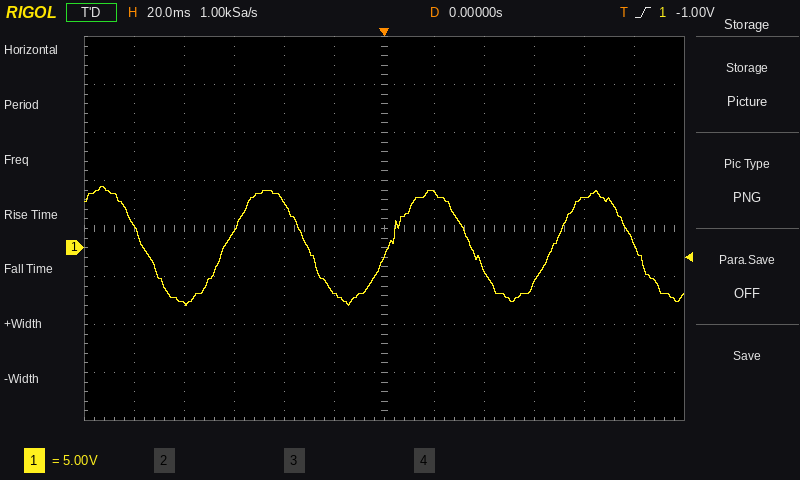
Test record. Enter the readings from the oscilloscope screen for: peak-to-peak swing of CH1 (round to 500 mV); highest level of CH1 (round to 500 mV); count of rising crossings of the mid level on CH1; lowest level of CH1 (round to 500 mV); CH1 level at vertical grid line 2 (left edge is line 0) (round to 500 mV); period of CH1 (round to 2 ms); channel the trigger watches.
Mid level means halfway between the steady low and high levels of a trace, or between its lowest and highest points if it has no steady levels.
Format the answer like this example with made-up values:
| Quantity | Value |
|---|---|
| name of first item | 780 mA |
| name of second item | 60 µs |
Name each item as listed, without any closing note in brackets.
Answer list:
| Quantity | Value |
|---|---|
| peak-to-peak swing of CH1 | 12.5 V |
| highest level of CH1 | 6.5 V |
| count of rising crossings of the mid level on CH1 | 3 |
| lowest level of CH1 | -6.0 V |
| CH1 level at vertical grid line 2 (left edge is line 0) | -6.0 V |
| period of CH1 | 66 ms |
| channel the trigger watches | CH1 |
